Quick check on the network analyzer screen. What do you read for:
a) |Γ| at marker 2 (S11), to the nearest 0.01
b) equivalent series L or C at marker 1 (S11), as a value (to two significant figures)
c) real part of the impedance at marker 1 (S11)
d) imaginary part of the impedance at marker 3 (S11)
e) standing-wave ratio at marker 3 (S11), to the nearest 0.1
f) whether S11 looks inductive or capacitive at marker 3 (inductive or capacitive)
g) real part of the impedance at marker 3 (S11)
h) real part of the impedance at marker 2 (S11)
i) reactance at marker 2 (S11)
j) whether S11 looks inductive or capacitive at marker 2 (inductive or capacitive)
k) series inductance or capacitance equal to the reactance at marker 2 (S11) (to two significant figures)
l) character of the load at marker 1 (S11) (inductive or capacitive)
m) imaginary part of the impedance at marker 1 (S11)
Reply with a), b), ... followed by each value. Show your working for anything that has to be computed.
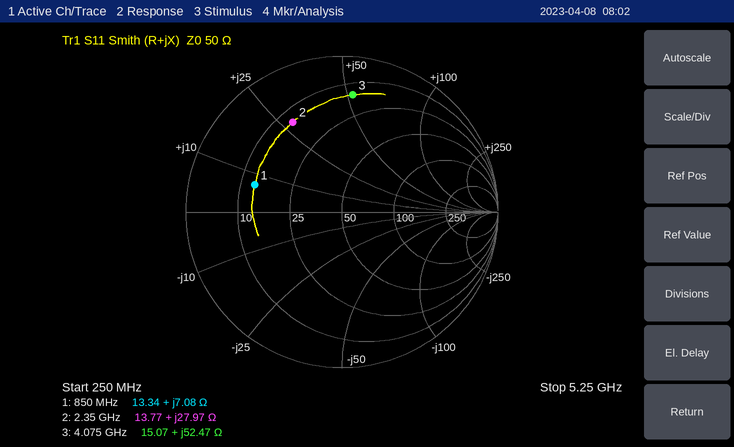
a) 0.66
b) L = 7.08 Ω/(2π × 850 MHz) ≈ 1.3 nH
c) 13.34 Ω
d) +52.47 Ω
e) 7.1
f) inductive
g) 15.07 Ω
h) 13.77 Ω
i) +27.97 Ω
j) inductive
k) L = 27.97 Ω/(2π × 2.35 GHz) ≈ 1.9 nH
l) inductive
m) +7.08 Ω
